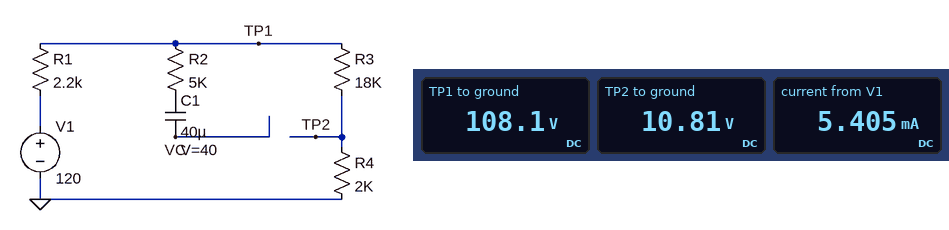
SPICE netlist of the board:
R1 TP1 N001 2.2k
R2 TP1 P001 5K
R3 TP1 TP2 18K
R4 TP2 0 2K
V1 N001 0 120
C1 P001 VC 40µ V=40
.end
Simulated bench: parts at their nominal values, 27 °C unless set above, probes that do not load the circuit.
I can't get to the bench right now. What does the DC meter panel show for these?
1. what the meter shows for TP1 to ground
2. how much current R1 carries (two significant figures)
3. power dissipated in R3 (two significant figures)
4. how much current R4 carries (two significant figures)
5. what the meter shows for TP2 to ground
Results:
108.1 V
5.4 mA
530 mW
5.4 mA
10.81 V
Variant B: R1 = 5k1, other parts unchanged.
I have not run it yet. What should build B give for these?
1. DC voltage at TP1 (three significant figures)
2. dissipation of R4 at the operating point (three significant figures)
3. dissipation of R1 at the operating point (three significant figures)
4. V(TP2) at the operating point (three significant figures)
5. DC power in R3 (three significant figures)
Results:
95.6 V
45.7 mW
117 mW
9.56 V
411 mW
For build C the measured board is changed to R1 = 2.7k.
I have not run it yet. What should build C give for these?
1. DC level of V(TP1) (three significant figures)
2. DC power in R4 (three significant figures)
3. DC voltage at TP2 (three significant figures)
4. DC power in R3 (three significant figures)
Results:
106 V
55.9 mW
10.6 V
503 mW
